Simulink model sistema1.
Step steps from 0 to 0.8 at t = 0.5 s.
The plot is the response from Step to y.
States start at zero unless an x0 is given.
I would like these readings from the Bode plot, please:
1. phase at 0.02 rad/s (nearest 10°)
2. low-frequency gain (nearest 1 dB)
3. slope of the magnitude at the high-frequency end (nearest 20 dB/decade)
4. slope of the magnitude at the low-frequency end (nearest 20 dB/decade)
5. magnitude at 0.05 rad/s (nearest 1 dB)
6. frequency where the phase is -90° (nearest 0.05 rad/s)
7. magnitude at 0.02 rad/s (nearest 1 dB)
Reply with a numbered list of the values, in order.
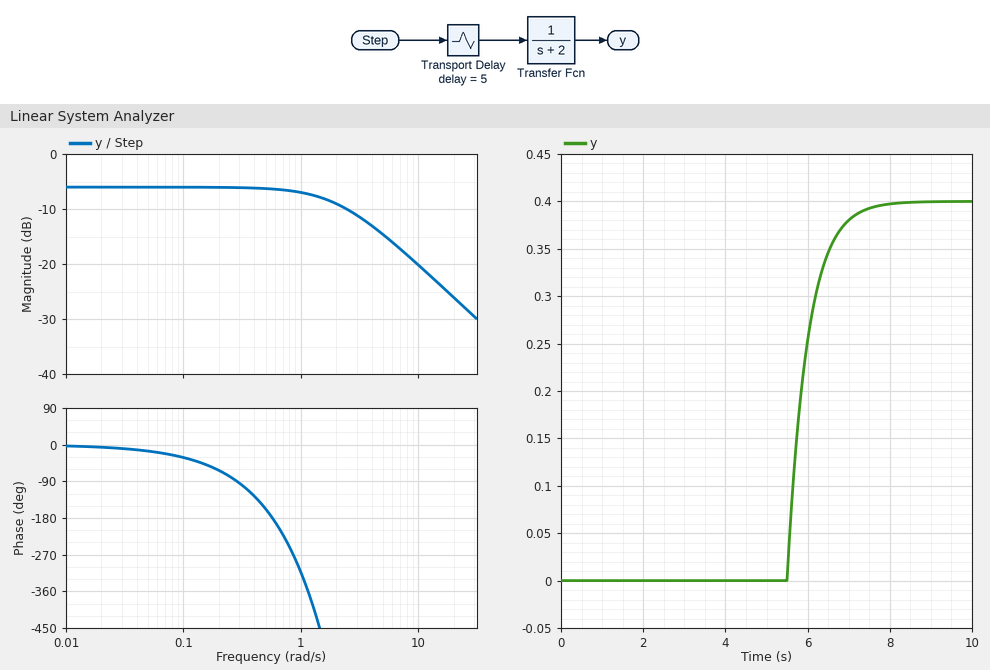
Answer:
1. -10°
2. -6 dB
3. -20 dB/decade
4. 0 dB/decade
5. -6 dB
6. 0.30 rad/s
7. -6 dB
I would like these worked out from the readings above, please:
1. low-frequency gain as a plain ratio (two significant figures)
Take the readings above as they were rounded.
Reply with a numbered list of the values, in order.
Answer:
1. 0.50
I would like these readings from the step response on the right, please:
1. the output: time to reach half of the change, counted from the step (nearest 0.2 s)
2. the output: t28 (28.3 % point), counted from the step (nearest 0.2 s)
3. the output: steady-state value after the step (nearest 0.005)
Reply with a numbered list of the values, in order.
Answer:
1. 5.4 s
2. 5.2 s
3. 0.400
